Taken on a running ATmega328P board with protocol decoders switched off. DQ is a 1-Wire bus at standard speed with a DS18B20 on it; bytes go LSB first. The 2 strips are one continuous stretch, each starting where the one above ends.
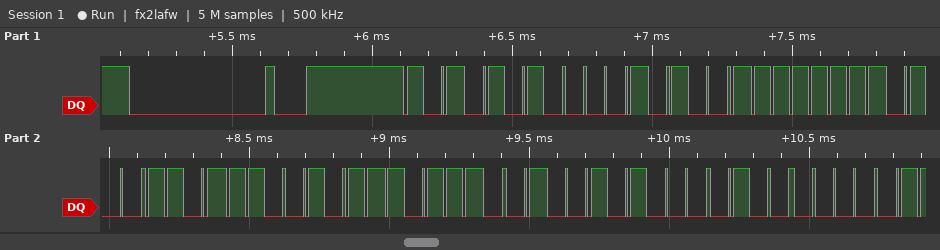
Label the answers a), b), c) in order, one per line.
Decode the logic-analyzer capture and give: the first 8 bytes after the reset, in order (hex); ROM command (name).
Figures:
a) 55 28 FF B2 D3 9D 14 02
b) Match ROM
